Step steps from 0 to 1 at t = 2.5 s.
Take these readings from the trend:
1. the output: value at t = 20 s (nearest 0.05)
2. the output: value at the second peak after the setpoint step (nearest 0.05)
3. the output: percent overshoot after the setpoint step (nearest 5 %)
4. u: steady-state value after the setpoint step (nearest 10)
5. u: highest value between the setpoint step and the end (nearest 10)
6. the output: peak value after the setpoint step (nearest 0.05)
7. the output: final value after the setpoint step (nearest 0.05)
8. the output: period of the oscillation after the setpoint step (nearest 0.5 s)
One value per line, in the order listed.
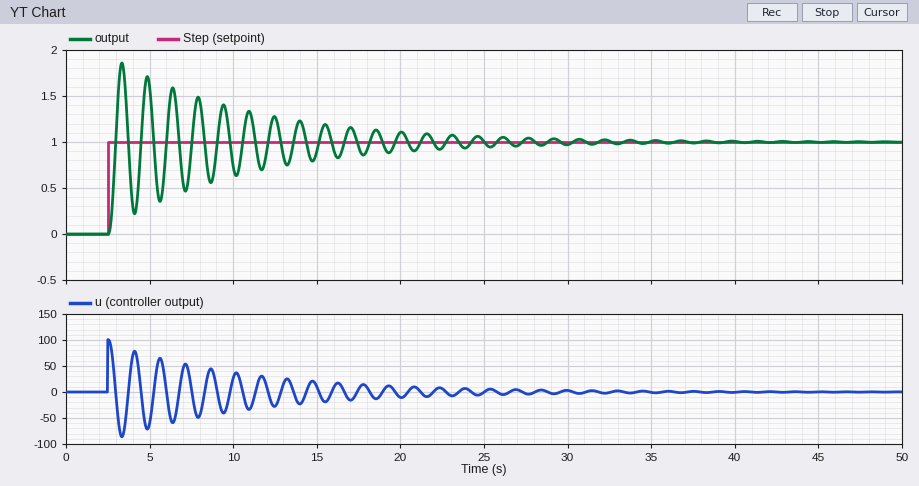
1.10
1.70
85 %
0
100
1.85
1.00
1.5 s
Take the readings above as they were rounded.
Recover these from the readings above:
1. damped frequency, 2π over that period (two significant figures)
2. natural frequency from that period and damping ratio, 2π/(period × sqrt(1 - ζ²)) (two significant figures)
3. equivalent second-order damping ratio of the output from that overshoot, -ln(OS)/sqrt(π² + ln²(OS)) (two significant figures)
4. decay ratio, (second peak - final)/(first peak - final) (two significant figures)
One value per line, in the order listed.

4.2 rad/s
4.2 rad/s
0.052
0.82
